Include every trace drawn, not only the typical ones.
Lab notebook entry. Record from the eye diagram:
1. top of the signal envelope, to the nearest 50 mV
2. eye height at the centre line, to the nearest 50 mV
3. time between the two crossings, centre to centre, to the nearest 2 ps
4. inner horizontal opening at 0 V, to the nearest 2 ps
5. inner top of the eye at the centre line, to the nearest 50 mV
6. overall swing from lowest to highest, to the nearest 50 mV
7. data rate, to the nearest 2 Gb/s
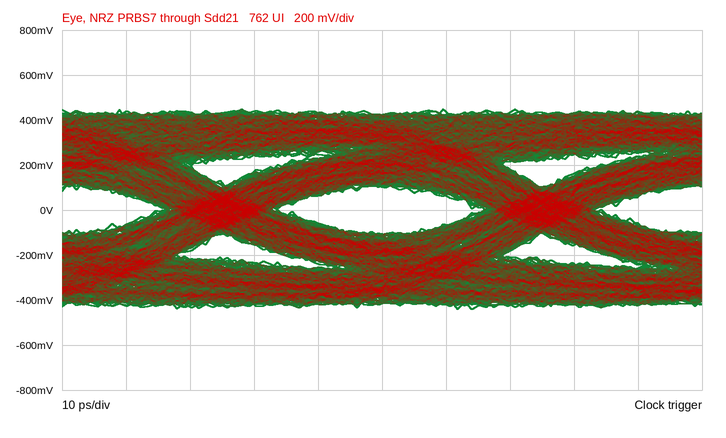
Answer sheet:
450 mV
200 mV
50 ps
32 ps
100 mV
900 mV
20 Gb/s
